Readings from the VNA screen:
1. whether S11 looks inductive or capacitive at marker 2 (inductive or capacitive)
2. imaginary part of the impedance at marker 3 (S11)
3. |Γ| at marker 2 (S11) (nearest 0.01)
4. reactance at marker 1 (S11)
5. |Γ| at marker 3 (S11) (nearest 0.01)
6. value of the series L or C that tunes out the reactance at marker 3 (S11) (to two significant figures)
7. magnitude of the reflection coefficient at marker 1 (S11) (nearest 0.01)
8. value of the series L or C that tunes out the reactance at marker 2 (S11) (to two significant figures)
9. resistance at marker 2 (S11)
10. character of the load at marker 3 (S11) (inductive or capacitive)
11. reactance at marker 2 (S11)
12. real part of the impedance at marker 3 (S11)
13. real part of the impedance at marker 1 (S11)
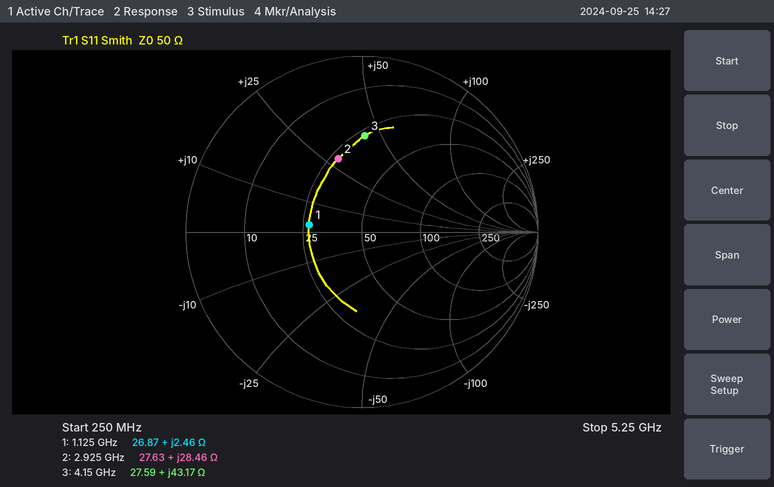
inductive
+43.17 Ω
0.44
+2.46 Ω
0.55
890 fF
0.30
1.9 pF
27.63 Ω
inductive
+28.46 Ω
27.59 Ω
26.87 Ω
